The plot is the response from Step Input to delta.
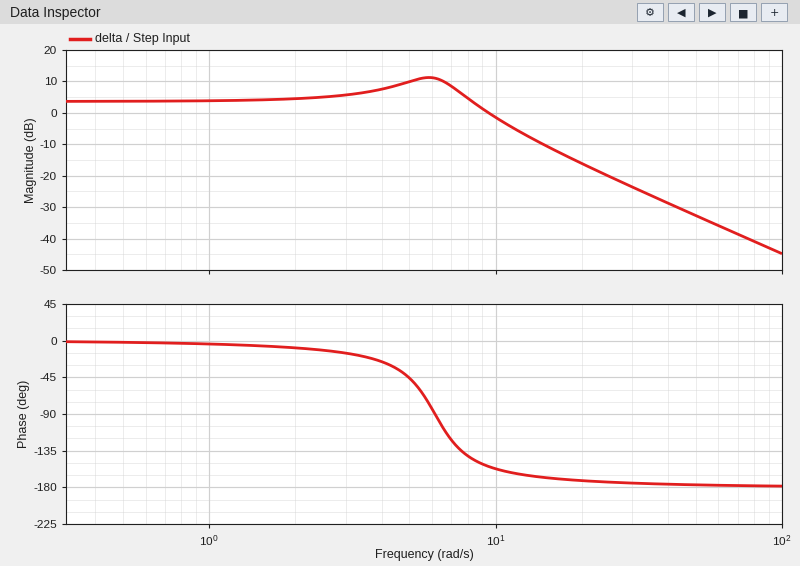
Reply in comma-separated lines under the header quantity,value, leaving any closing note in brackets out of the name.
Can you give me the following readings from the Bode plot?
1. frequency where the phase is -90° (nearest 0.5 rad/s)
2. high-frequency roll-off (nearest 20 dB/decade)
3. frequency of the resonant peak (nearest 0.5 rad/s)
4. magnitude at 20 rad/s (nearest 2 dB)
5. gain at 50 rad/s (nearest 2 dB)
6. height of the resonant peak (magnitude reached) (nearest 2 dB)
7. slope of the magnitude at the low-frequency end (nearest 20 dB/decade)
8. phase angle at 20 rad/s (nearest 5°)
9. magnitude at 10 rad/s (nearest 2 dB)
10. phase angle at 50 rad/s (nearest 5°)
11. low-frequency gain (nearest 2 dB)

quantity,value
frequency where the phase is -90°,6.0 rad/s
high-frequency roll-off,-40 dB/decade
frequency of the resonant peak,6.0 rad/s
magnitude at 20 rad/s,-16 dB
gain at 50 rad/s,-32 dB
height of the resonant peak (magnitude reached),12 dB
slope of the magnitude at the low-frequency end,0 dB/decade
phase angle at 20 rad/s,-170°
magnitude at 10 rad/s,-2 dB
phase angle at 50 rad/s,-175°
low-frequency gain,4 dB
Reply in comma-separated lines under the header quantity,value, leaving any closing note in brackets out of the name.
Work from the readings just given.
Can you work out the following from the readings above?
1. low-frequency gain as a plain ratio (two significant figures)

quantity,value
low-frequency gain as a plain ratio,1.6
